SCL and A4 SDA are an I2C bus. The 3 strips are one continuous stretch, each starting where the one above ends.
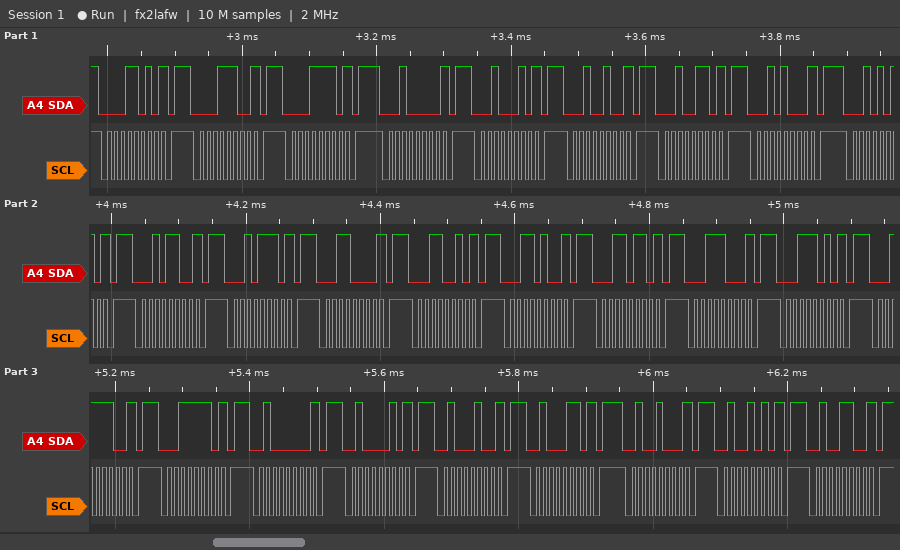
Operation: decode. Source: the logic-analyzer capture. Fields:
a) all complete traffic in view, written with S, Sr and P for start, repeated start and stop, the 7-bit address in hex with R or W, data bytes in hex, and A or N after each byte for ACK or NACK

S 0DW N P S 0EW N P S 0FW N P S 10W N P S 11W N P S 12W N P S 13W N P S 14W N P S 15W N P S 16W N P S 17W N P S 18W N P S 19W N P S 1AW N P S 1BW N P S 1CW N P S 1DW N P S 1EW N P S 1FW N P S 20W N P S 21W N P S 22W N P S 23W N P S 24W N P S 25W N P S 26W N P
